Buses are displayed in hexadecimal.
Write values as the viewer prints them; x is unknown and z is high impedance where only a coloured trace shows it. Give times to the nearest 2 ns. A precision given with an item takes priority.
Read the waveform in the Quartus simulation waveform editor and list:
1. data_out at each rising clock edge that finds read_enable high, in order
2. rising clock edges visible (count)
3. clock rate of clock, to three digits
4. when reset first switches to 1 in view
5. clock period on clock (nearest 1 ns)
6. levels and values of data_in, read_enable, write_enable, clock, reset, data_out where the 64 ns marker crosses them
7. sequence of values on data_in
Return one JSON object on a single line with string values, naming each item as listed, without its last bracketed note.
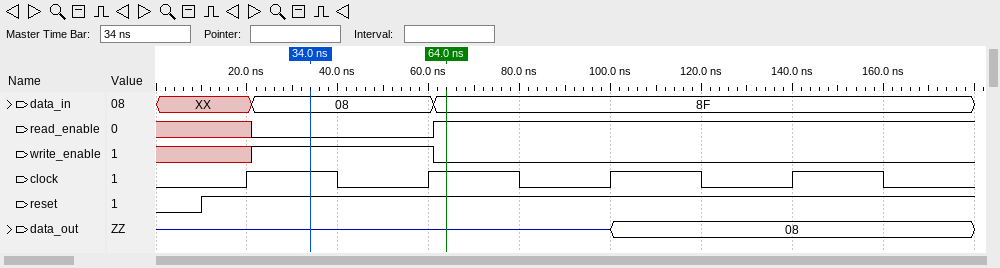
{"data_out at each rising clock edge that finds read_enable high, in order": "z, 08", "rising clock edges visible": "4", "clock rate of clock, to three digits": "25.0 MHz", "when reset first switches to 1 in view": "10 ns", "clock period on clock": "40 ns", "levels and values of data_in, read_enable, write_enable, clock, reset, data_out where the 64 ns marker crosses them": "data_in=8F, read_enable=1, write_enable=0, clock=1, reset=1, data_out=z", "sequence of values on data_in": "XX, 08, 8F"}
